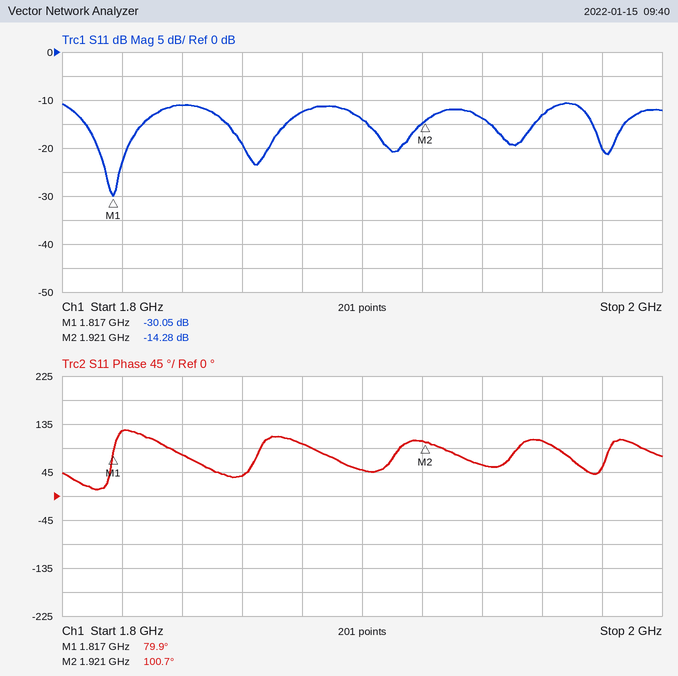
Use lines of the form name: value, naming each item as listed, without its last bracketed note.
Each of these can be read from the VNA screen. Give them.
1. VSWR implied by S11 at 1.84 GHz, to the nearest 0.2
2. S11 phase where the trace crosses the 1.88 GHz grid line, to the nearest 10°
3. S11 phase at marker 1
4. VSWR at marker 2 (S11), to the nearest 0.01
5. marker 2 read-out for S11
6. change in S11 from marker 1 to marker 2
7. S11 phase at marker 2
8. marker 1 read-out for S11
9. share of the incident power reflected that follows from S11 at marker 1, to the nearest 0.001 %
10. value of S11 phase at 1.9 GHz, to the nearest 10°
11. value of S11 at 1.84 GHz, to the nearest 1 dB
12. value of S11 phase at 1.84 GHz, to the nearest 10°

VSWR implied by S11 at 1.84 GHz, to the nearest 0.2: 1.8
S11 phase where the trace crosses the 1.88 GHz grid line, to the nearest 10°: 100°
S11 phase at marker 1: 79.9°
VSWR at marker 2 (S11), to the nearest 0.01: 1.48
marker 2 read-out for S11: -14.28 dB
change in S11 from marker 1 to marker 2: 15.77 dB
S11 phase at marker 2: 100.7°
marker 1 read-out for S11: -30.05 dB
share of the incident power reflected that follows from S11 at marker 1, to the nearest 0.001 %: 0.099 %
value of S11 phase at 1.9 GHz, to the nearest 10°: 50°
value of S11 at 1.84 GHz, to the nearest 1 dB: -11 dB
value of S11 phase at 1.84 GHz, to the nearest 10°: 80°
